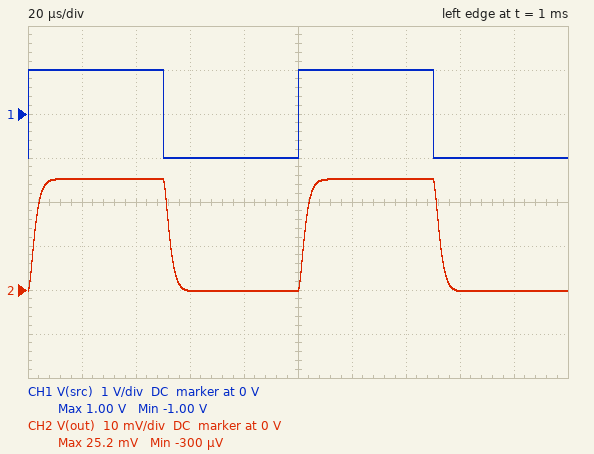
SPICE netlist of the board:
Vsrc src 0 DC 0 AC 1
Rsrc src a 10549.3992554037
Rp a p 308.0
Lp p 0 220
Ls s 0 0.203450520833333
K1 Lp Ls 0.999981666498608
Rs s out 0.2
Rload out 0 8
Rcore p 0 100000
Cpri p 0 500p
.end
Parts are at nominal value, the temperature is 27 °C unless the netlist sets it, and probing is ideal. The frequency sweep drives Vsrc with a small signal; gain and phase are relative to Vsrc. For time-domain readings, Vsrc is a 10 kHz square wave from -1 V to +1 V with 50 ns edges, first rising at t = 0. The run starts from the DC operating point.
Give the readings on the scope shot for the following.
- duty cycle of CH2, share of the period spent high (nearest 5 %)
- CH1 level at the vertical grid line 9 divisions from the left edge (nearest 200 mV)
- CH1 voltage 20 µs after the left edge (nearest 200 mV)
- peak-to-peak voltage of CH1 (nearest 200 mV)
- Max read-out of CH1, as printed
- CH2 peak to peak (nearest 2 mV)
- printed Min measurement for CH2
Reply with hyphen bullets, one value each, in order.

- 50 %
- -1.0 V
- 1.0 V
- 2.0 V
- 1.00 V
- 26 mV
- -300 µV
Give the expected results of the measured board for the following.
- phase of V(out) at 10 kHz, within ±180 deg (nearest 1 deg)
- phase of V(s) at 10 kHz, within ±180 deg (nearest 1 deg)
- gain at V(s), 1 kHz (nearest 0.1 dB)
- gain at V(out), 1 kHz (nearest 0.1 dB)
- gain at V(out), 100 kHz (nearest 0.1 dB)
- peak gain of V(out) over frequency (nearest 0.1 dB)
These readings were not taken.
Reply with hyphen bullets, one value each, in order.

- -10 deg
- -10 deg
- -37.7 dB
- -37.9 dB
- -42.7 dB
- -37.9 dB
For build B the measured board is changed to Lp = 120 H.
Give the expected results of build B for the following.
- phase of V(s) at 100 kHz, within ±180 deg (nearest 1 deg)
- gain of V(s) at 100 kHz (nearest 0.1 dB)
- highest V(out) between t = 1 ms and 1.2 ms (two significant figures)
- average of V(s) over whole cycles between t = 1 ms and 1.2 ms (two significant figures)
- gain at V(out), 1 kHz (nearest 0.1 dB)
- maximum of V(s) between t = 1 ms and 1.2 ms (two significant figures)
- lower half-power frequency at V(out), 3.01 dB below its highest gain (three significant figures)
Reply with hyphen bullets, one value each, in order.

- -71 deg
- -40.3 dB
- 24 mV
- 12 mV
- -38.4 dB
- 25 mV
- 4.29 Hz
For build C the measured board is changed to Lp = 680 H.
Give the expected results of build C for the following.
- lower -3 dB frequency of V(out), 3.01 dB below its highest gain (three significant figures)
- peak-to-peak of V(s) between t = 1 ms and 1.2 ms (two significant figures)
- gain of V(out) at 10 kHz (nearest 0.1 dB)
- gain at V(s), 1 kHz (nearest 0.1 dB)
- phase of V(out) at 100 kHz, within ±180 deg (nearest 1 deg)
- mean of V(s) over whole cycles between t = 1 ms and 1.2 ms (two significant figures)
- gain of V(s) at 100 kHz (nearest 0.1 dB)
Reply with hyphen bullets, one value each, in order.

- 1.69 Hz
- 23 mV
- -39.2 dB
- -38.8 dB
- -96 deg
- 11 mV
- -47.4 dB
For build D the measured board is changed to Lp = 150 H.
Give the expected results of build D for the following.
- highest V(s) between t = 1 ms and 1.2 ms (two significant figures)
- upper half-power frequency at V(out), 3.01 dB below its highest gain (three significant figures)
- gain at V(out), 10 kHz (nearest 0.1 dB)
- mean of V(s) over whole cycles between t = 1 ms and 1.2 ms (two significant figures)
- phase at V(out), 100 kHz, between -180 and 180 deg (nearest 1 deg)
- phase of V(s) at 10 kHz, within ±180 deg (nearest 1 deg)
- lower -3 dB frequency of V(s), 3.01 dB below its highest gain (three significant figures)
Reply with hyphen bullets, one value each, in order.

- 25 mV
- 98.4 kHz
- -38.2 dB
- 12 mV
- -77 deg
- -8 deg
- 3.97 Hz
